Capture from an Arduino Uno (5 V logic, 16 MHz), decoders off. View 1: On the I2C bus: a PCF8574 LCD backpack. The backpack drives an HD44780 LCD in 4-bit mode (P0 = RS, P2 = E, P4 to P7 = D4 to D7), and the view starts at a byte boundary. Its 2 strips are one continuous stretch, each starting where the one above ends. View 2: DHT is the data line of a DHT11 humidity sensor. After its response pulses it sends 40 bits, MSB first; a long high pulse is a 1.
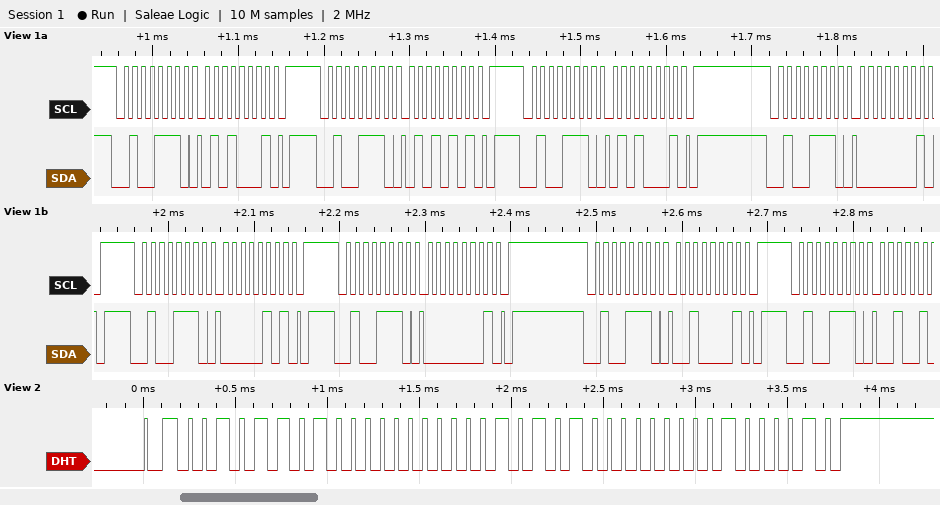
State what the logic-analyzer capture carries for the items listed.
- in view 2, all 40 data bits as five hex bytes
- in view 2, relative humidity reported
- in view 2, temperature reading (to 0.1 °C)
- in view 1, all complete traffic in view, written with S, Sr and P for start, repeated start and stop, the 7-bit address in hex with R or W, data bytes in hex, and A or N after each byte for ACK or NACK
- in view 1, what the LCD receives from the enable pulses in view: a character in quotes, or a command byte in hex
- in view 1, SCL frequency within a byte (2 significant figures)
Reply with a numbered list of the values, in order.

1. 2D 00 15 00 42
2. 45 %
3. 21.0 °C
4. S 27W A 51 A P S 27W A 55 A P S 27W A 51 A P S 27W A 01 A P S 27W A 05 A P S 27W A 01 A P S 27W A 21 A P S 27W A
5. 'P'
6. 100 kHz
